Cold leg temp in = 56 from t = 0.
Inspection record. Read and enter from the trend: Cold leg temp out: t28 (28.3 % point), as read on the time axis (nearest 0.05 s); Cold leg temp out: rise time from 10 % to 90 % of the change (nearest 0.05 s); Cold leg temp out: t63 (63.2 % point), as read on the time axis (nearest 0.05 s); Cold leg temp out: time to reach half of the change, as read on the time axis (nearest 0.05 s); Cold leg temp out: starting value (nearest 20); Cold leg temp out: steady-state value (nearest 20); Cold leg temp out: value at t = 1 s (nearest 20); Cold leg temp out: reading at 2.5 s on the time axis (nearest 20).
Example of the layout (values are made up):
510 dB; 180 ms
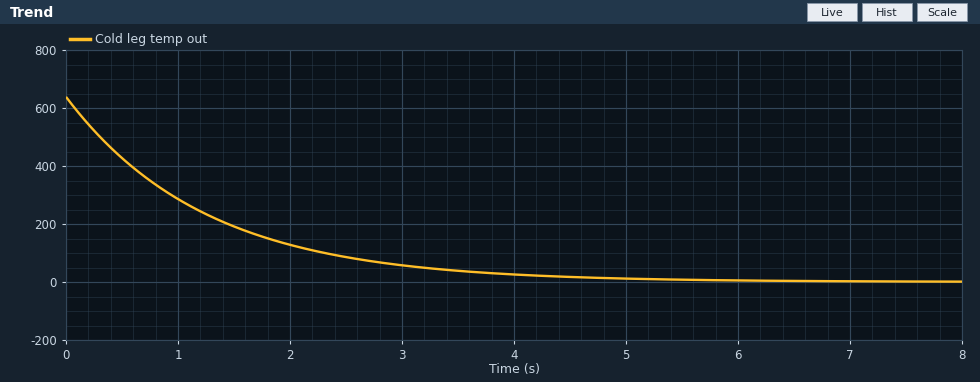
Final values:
0.40 s; 2.75 s; 1.25 s; 0.85 s; 640; 0; 280; 80
